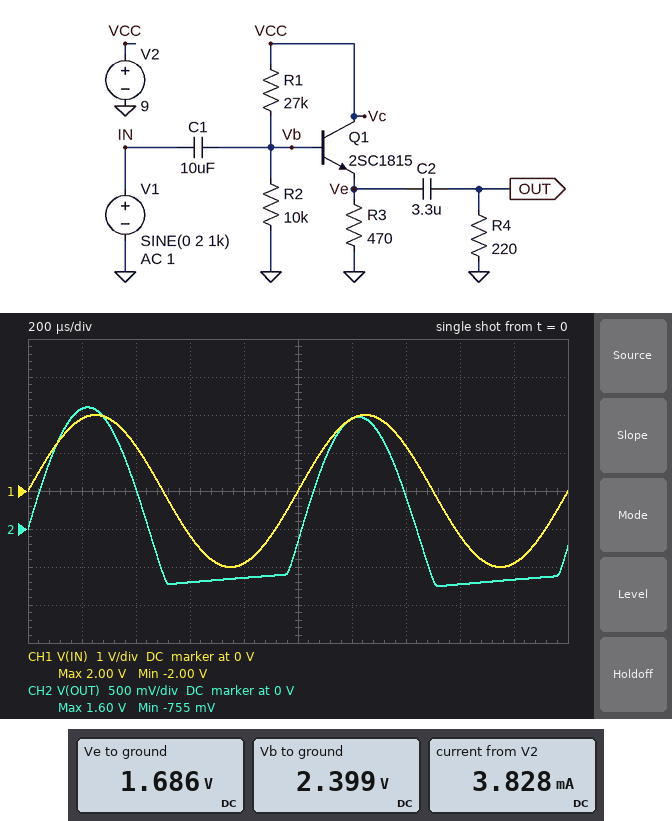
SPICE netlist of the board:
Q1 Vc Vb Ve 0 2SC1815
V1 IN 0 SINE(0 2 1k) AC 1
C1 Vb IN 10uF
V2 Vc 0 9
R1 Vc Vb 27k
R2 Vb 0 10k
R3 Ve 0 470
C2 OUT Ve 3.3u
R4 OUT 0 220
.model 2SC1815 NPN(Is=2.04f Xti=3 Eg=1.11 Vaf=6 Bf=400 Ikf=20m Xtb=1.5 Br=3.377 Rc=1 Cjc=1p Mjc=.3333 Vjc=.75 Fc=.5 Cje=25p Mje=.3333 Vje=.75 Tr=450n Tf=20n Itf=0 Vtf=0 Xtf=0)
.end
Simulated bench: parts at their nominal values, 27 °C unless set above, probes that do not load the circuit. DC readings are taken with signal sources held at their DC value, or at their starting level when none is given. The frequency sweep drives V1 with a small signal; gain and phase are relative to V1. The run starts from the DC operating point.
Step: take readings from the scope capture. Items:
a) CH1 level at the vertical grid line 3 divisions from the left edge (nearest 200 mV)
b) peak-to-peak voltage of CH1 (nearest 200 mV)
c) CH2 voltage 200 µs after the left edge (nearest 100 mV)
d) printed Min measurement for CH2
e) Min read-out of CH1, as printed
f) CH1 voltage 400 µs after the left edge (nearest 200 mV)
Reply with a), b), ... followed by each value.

a) -1.2 V
b) 4.0 V
c) 1.6 V
d) -755 mV
e) -2.00 V
f) 1.2 V
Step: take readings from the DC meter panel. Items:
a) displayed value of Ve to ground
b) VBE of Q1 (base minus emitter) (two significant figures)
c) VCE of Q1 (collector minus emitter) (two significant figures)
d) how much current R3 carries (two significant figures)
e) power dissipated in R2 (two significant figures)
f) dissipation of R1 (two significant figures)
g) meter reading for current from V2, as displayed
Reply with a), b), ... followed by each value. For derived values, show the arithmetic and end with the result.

a) 1.686 V
b) 2.399 V - 1.686 V = 710 mV
c) 9 V - 1.686 V = 7.3 V
d) (1.686 V) / 470 Ω = 3.6 mA
e) (2.399 V)^2 / 10 kΩ = 580 µW
f) (9 V - 2.399 V)^2 / 27 kΩ = 1.6 mW
g) 3.828 mA
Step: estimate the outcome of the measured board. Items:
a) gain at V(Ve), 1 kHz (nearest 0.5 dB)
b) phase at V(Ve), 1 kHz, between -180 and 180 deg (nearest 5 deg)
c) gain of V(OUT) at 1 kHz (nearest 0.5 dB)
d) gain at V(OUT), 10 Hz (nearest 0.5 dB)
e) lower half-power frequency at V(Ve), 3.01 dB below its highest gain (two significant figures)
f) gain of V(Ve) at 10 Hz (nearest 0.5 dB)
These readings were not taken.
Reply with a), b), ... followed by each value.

a) -0.5 dB
b) 0 deg
c) -0.5 dB
d) -27.0 dB
e) 2.2 Hz
f) -0.5 dB
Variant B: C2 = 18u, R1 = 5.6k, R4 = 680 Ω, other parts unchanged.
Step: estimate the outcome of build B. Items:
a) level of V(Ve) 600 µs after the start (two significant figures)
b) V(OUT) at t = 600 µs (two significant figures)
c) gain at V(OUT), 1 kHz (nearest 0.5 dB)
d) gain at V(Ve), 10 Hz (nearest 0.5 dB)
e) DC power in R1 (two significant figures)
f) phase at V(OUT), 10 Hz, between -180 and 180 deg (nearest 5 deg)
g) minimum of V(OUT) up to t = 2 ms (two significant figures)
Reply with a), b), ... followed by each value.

a) 3.8 V
b) -1.2 V
c) 0 dB
d) -1.0 dB
e) 2.0 mW
f) 75 deg
g) -2.0 V
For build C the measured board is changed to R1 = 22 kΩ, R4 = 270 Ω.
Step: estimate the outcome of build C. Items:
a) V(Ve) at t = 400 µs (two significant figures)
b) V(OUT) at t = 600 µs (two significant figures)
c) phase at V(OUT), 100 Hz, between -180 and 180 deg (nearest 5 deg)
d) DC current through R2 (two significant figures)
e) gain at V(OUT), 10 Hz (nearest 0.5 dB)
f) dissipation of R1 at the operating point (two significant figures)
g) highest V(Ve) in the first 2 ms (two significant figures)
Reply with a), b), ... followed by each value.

a) 3.2 V
b) -910 mV
c) 60 deg
d) 280 µA
e) -25.5 dB
f) 1.8 mW
g) 4.0 V
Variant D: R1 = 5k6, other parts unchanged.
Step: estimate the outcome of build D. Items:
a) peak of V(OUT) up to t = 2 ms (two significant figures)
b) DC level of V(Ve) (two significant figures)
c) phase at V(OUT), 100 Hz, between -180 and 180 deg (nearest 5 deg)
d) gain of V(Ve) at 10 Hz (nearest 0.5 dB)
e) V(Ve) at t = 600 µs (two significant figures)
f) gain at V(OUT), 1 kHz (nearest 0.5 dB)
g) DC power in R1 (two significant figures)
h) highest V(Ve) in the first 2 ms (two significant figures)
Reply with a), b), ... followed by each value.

a) 1.8 V
b) 4.9 V
c) 70 deg
d) -1.0 dB
e) 3.8 V
f) -0.5 dB
g) 2.0 mW
h) 6.9 V
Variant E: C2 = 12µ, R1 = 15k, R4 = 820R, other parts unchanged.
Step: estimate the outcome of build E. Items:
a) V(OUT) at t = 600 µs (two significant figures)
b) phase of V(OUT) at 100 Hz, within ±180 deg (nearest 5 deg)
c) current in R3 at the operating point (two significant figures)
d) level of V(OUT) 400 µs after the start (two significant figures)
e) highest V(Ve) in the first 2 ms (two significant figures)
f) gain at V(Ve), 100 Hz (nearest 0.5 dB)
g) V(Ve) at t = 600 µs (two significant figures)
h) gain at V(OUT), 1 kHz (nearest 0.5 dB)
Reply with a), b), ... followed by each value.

a) -1.2 V
b) 10 deg
c) 6.0 mA
d) 1.1 V
e) 4.8 V
f) 0 dB
g) 1.7 V
h) 0 dB
